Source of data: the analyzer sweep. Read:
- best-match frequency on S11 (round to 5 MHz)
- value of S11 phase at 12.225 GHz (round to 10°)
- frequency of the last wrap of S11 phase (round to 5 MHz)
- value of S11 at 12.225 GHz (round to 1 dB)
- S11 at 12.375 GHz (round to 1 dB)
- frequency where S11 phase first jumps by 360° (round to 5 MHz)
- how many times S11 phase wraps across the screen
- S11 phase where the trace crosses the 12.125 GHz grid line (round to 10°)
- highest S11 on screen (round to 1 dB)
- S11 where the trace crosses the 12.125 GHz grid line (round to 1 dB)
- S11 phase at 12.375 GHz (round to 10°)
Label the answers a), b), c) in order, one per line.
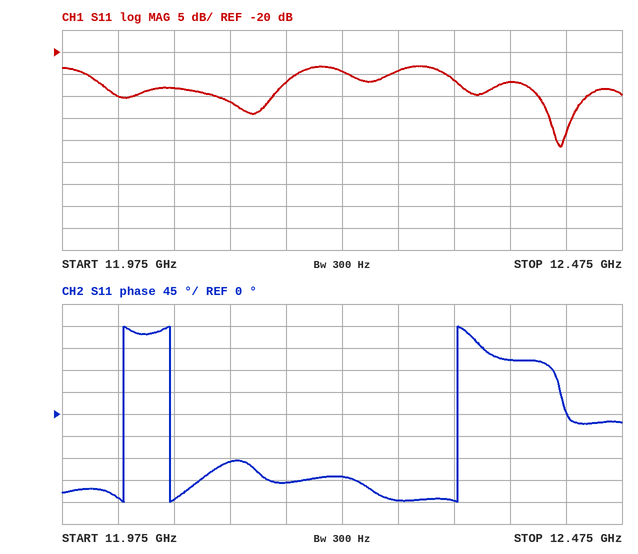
a) 12.420 GHz
b) -130°
c) 12.330 GHz
d) -24 dB
e) -27 dB
f) 12.030 GHz
g) 3
h) -100°
i) -23 dB
j) -31 dB
k) 110°
